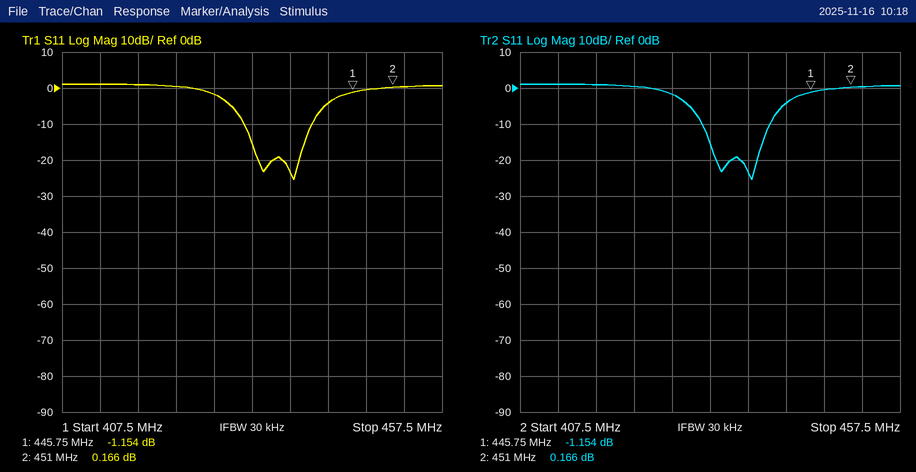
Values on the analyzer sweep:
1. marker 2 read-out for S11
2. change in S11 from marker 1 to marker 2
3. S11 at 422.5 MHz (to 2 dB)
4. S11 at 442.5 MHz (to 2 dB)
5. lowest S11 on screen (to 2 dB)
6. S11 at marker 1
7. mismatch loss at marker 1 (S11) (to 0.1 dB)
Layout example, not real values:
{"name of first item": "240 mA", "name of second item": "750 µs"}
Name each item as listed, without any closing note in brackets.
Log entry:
{"marker 2 read-out for S11": "0.166 dB", "change in S11 from marker 1 to marker 2": "1.320 dB", "S11 at 422.5 MHz": "0 dB", "S11 at 442.5 MHz": "-4 dB", "lowest S11 on screen": "-26 dB", "S11 at marker 1": "-1.154 dB", "mismatch loss at marker 1 (S11)": "6.3 dB"}
